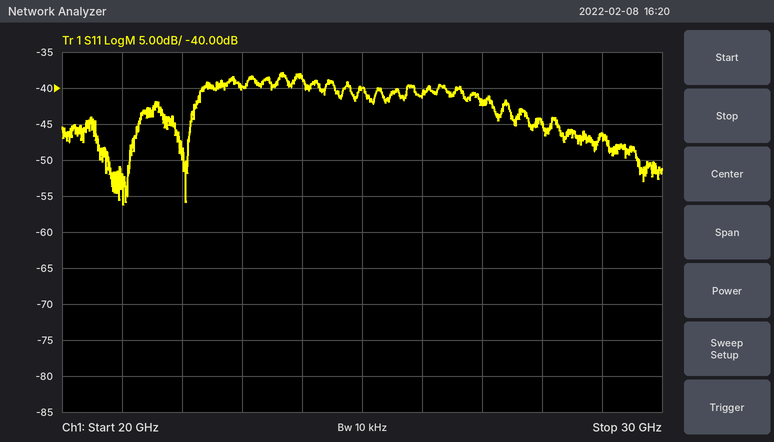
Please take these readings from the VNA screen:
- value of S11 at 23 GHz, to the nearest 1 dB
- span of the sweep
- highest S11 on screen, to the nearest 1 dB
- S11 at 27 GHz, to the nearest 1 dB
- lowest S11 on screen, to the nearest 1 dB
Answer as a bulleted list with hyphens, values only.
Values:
- -40 dB
- 10 GHz
- -38 dB
- -42 dB
- -56 dB
